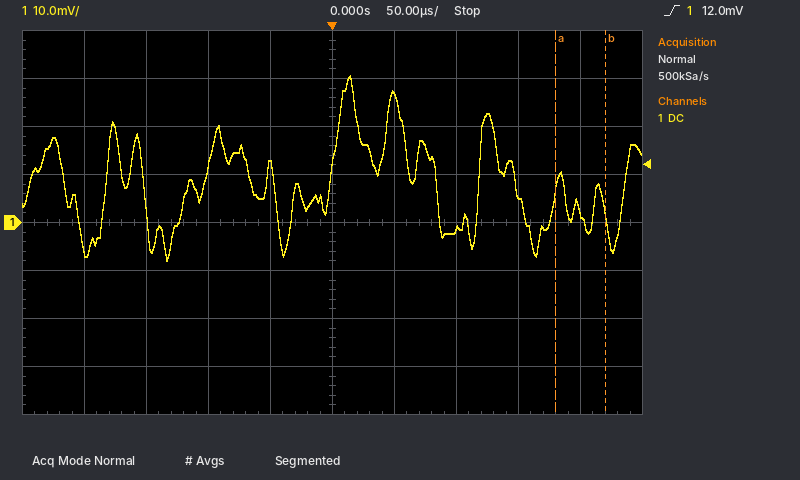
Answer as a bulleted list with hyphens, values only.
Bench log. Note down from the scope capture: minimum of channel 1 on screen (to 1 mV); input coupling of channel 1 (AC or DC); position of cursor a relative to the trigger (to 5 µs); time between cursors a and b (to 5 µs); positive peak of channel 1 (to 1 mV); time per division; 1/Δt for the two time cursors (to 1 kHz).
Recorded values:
- -8 mV
- DC
- +180 µs
- 40 µs
- 31 mV
- 50 µs
- 25 kHz
